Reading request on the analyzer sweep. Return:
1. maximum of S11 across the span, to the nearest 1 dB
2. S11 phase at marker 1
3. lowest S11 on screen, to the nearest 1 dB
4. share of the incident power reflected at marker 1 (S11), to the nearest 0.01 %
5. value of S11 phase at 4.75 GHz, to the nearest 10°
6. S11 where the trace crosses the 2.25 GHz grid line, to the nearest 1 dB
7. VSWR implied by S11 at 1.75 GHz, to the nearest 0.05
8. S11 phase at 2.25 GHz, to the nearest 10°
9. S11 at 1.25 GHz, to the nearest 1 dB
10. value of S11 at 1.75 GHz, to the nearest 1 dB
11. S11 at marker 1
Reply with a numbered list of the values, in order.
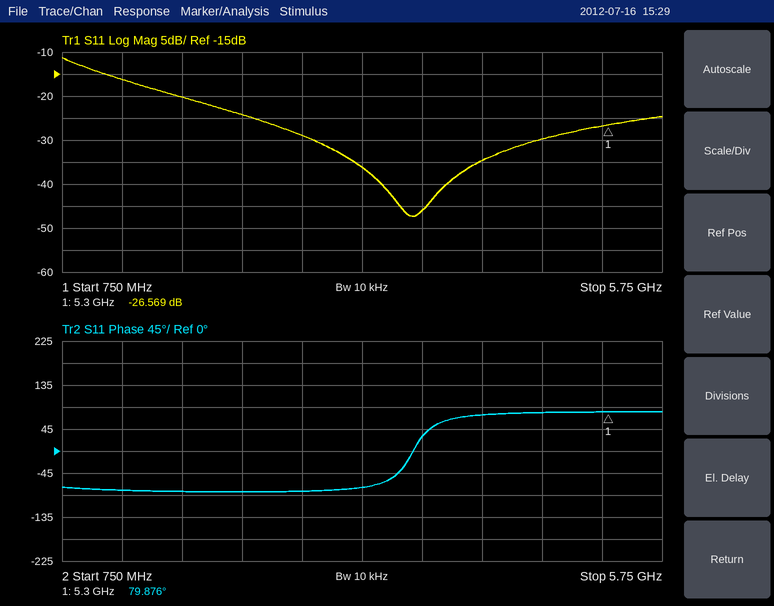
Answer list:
1. -11 dB
2. 79.876°
3. -47 dB
4. 0.22 %
5. 80°
6. -24 dB
7. 1.20
8. -80°
9. -16 dB
10. -20 dB
11. -26.569 dB
